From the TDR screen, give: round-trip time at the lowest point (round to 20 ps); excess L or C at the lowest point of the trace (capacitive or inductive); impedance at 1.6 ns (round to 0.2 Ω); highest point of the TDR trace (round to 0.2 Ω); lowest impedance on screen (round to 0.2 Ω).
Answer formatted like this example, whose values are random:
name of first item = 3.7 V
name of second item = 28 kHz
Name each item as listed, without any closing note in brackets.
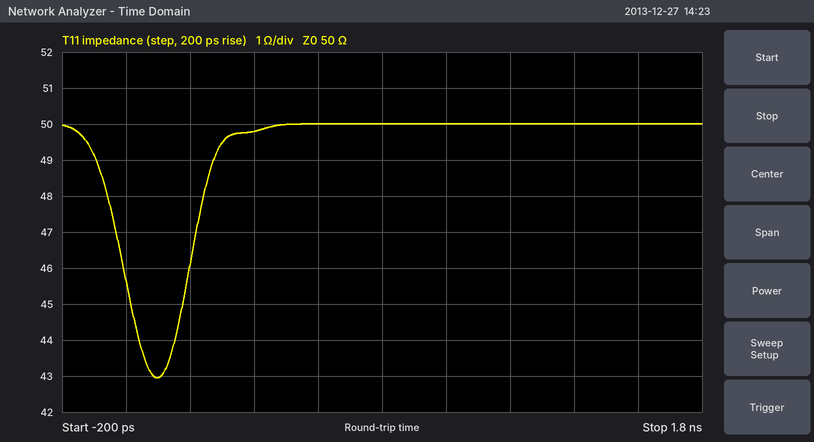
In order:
round-trip time at the lowest point = 100 ps
excess L or C at the lowest point of the trace = capacitive
impedance at 1.6 ns = 50.0 Ω
highest point of the TDR trace = 50.0 Ω
lowest impedance on screen = 43.0 Ω
